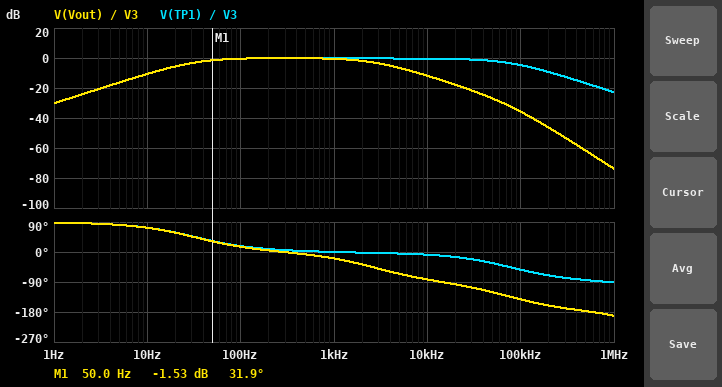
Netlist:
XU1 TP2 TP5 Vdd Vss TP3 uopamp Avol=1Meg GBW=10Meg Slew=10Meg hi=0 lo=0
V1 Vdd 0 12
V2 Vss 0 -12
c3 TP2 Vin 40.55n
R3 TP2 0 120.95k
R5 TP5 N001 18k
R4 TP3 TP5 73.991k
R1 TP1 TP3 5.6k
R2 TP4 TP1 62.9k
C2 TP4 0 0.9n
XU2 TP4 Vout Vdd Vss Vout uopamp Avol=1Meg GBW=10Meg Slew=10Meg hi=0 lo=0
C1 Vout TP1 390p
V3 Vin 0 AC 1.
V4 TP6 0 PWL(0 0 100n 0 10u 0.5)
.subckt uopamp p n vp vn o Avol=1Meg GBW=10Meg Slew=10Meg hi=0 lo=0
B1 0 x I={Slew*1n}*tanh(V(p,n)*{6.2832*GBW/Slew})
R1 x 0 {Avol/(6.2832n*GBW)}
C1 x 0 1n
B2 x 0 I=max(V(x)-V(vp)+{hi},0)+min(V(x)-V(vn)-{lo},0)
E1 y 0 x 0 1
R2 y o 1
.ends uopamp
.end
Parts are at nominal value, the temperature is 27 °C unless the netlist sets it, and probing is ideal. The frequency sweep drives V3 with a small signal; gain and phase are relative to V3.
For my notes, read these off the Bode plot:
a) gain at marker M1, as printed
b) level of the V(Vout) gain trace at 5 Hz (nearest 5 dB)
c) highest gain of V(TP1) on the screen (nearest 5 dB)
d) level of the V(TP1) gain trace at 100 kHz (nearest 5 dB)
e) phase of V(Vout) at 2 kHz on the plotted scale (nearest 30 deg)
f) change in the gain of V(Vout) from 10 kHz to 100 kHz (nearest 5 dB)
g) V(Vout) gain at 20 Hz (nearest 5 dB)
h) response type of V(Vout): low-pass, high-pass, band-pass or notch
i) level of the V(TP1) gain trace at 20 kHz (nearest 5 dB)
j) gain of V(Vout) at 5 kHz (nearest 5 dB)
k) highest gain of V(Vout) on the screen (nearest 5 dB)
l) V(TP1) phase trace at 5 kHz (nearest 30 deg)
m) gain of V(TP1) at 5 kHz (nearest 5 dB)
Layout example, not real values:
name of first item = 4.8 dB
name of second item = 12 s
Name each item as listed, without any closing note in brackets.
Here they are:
gain at marker M1, as printed = -1.53 dB
level of the V(Vout) gain trace at 5 Hz = -15 dB
highest gain of V(TP1) on the screen = 0 dB
level of the V(TP1) gain trace at 100 kHz = -5 dB
phase of V(Vout) at 2 kHz on the plotted scale = -30 deg
change in the gain of V(Vout) from 10 kHz to 100 kHz = -25 dB
V(Vout) gain at 20 Hz = -5 dB
response type of V(Vout): low-pass, high-pass, band-pass or notch = band-pass
level of the V(TP1) gain trace at 20 kHz = 0 dB
gain of V(Vout) at 5 kHz = -5 dB
highest gain of V(Vout) on the screen = 0 dB
V(TP1) phase trace at 5 kHz = 0 deg
gain of V(TP1) at 5 kHz = 0 dB
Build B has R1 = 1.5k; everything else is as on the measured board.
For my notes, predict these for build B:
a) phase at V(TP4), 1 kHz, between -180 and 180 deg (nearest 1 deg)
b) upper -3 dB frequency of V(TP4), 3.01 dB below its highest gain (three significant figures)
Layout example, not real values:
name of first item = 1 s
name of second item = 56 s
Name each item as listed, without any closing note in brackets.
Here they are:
phase at V(TP4), 1 kHz, between -180 and 180 deg = -18 deg
upper -3 dB frequency of V(TP4), 3.01 dB below its highest gain = 2.84 kHz
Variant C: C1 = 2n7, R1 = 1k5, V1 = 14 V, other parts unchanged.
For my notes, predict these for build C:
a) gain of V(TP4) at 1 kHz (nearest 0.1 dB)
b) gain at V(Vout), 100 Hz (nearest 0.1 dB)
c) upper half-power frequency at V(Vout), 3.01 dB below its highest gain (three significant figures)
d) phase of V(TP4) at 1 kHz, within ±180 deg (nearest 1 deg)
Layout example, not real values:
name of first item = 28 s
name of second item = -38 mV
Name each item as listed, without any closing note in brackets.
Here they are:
gain of V(TP4) at 1 kHz = -0.5 dB
gain at V(Vout), 100 Hz = -0.4 dB
upper half-power frequency at V(Vout), 3.01 dB below its highest gain = 3.01 kHz
phase of V(TP4) at 1 kHz, within ±180 deg = -18 deg
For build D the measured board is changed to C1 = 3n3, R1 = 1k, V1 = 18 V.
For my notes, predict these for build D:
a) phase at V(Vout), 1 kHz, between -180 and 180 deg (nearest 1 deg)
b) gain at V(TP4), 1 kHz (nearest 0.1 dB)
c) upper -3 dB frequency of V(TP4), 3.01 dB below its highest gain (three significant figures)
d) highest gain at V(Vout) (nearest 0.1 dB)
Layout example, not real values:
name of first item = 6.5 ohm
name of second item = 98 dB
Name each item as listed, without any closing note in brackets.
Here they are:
phase at V(Vout), 1 kHz, between -180 and 180 deg = -18 deg
gain at V(TP4), 1 kHz = -0.5 dB
upper -3 dB frequency of V(TP4), 3.01 dB below its highest gain = 3.00 kHz
highest gain at V(Vout) = -0.1 dB
